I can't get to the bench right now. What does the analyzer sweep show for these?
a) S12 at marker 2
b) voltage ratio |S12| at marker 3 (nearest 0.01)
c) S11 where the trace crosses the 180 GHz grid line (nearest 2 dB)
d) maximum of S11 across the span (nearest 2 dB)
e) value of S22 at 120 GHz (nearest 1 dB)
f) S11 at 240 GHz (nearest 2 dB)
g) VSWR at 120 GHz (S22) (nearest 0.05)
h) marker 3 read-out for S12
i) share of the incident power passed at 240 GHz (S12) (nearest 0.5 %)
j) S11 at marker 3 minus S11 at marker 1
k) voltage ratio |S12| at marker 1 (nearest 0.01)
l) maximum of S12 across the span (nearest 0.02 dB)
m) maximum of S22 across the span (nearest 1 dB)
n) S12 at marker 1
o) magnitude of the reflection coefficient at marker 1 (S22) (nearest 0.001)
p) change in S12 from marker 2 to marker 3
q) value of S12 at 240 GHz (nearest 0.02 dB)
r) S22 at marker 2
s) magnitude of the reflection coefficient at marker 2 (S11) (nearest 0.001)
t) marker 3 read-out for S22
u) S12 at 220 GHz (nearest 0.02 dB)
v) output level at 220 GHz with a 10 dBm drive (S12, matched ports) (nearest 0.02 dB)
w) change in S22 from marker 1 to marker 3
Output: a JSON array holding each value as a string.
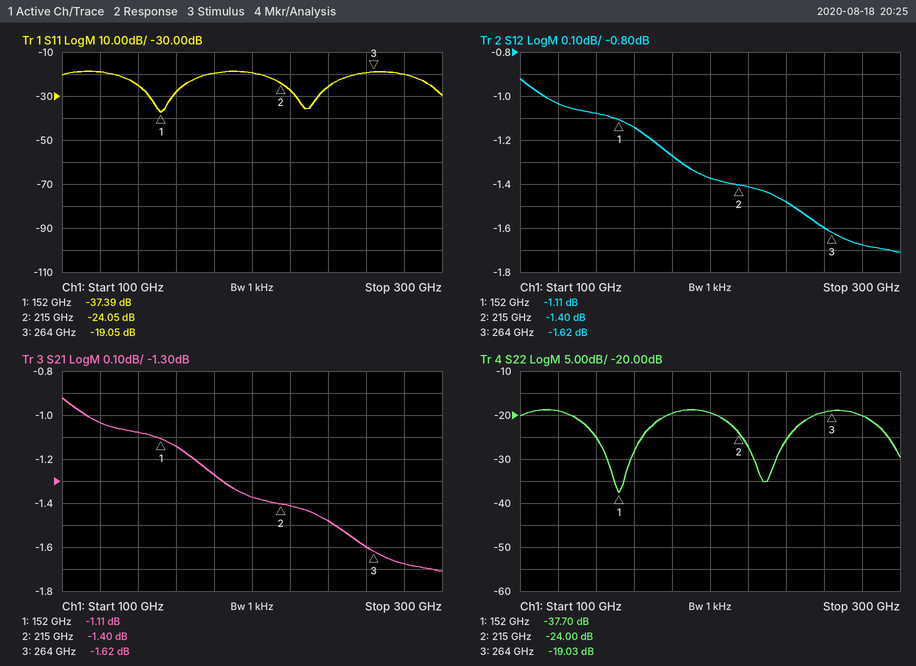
["-1.40 dB", "0.83", "-20 dB", "-18 dB", "-19 dB", "-26 dB", "1.25", "-1.62 dB", "71.0 %", "18.34 dB", "0.88", "-0.92 dB", "-19 dB", "-1.11 dB", "0.013", "-0.22 dB", "-1.48 dB", "-24.00 dB", "0.063", "-19.03 dB", "-1.42 dB", "8.58 dBm", "18.67 dB"]
